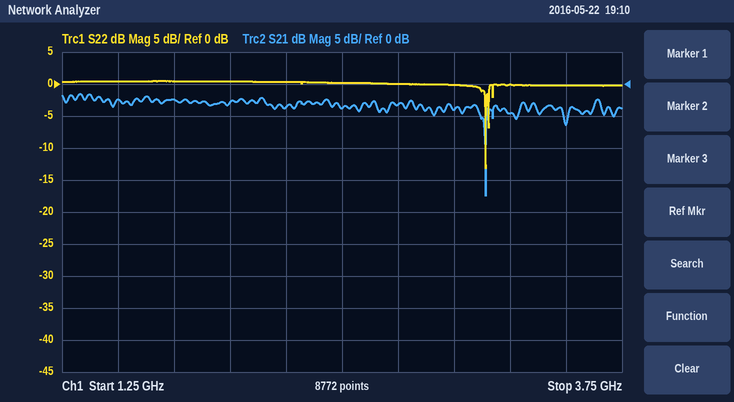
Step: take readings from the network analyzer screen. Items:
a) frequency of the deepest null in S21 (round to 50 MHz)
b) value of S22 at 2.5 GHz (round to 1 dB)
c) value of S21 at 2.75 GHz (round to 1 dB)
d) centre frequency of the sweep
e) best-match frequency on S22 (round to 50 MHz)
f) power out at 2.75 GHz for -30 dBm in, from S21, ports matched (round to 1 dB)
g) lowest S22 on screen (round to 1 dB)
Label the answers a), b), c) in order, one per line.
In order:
a) 3.15 GHz
b) 0 dB
c) -3 dB
d) 2.5 GHz
e) 3.15 GHz
f) -33 dBm
g) -13 dB
